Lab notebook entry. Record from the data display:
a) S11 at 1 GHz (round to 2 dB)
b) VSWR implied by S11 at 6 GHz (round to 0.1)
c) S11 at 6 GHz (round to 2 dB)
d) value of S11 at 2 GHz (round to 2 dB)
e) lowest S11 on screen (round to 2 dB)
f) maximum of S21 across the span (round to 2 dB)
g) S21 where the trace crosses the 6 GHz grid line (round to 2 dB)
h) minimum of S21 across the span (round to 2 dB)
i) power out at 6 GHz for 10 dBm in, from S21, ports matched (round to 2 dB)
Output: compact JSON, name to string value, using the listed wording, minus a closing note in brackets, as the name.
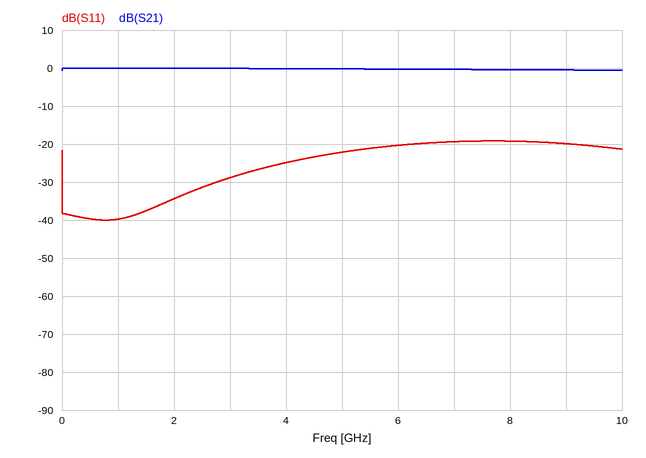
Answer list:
{"S11 at 1 GHz": "-40 dB", "VSWR implied by S11 at 6 GHz": "1.2", "S11 at 6 GHz": "-20 dB", "value of S11 at 2 GHz": "-34 dB", "lowest S11 on screen": "-40 dB", "maximum of S21 across the span": "0 dB", "S21 where the trace crosses the 6 GHz grid line": "0 dB", "minimum of S21 across the span": "0 dB", "power out at 6 GHz for 10 dBm in, from S21, ports matched": "10 dBm"}
